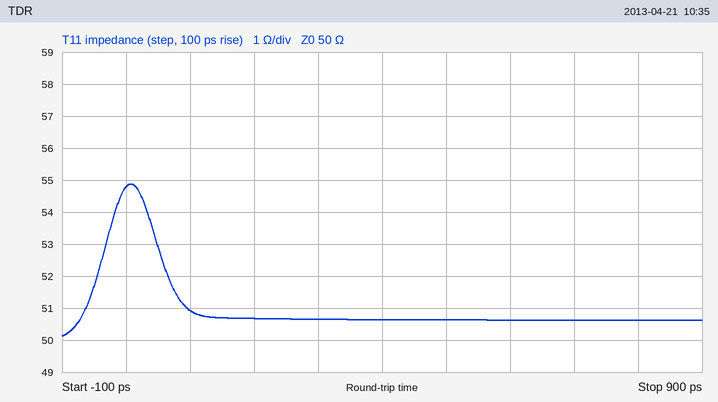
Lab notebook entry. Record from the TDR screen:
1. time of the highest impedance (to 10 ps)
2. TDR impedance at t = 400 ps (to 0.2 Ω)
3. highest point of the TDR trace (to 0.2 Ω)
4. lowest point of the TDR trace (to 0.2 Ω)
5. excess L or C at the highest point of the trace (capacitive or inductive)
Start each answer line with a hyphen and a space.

- 10 ps
- 50.6 Ω
- 54.8 Ω
- 50.2 Ω
- inductive
